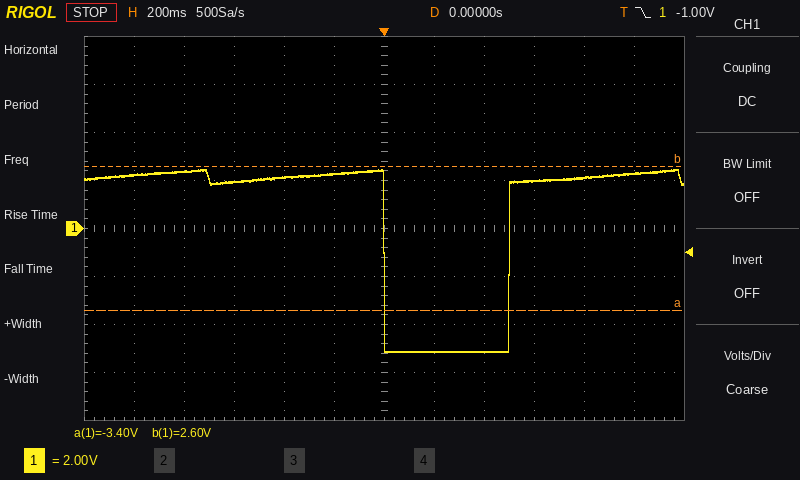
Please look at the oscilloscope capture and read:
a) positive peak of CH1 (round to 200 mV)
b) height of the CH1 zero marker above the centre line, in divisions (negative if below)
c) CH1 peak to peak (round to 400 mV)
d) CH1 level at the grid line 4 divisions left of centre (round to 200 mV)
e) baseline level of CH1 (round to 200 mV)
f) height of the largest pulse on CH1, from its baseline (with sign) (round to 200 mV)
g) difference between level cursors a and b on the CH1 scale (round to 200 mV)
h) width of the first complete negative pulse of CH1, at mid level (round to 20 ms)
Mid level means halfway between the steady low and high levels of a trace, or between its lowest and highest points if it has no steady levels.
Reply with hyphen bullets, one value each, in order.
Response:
- 2.4 V
- 0.0 div
- 7.6 V
- 2.4 V
- 2.2 V
- -7.2 V
- 6.0 V
- 500 ms
